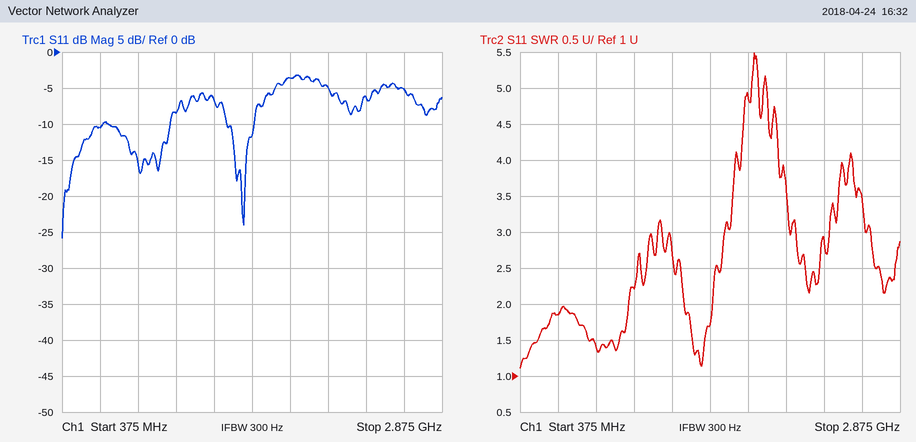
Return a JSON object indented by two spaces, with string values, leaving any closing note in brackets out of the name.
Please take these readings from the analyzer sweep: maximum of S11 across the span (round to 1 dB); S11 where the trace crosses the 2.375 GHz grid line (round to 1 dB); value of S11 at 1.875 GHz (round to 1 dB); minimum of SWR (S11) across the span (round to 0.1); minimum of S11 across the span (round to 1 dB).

{
  "maximum of S11 across the span": "-3 dB",
  "S11 where the trace crosses the 2.375 GHz grid line": "-6 dB",
  "value of S11 at 1.875 GHz": "-4 dB",
  "minimum of SWR (S11) across the span": "1.1",
  "minimum of S11 across the span": "-26 dB"
}
